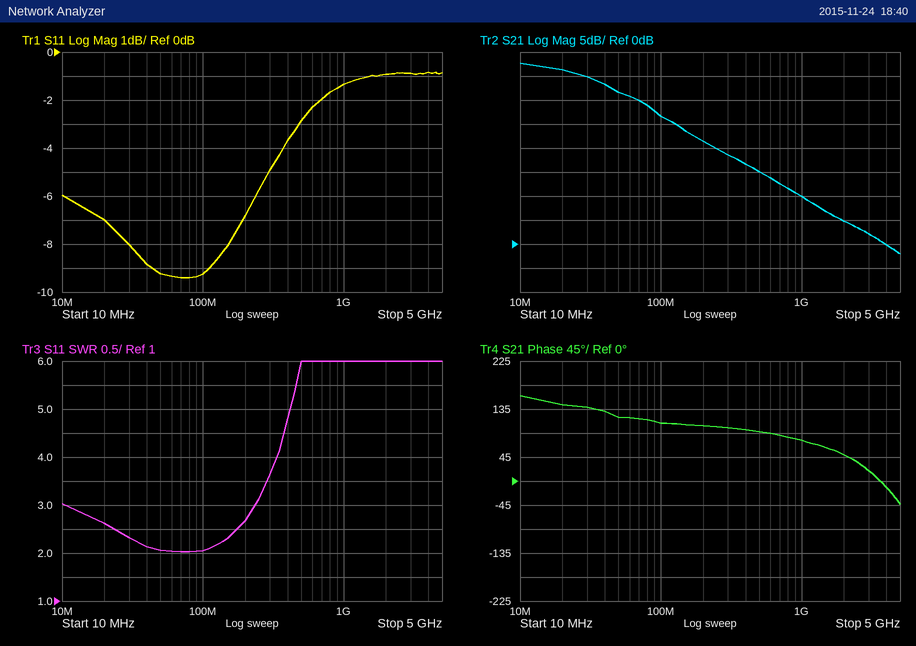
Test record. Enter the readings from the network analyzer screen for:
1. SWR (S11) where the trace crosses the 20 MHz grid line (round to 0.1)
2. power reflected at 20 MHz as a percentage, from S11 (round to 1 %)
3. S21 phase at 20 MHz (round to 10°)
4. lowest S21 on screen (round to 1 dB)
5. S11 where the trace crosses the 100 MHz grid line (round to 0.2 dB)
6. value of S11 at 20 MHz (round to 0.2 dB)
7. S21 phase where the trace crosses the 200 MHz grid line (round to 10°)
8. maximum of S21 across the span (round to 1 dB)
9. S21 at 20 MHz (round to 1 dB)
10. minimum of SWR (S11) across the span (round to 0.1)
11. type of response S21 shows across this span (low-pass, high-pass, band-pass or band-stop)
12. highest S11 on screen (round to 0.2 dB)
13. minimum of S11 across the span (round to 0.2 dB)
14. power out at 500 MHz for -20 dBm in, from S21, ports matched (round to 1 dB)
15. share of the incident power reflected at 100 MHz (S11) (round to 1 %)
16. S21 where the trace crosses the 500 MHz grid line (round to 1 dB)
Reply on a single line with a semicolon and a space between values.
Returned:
2.6; 20 %; 140°; -2 dB; -9.2 dB; -7.0 dB; 100°; 38 dB; 36 dB; 2.0; low-pass; -0.8 dB; -9.4 dB; -5 dBm; 12 %; 15 dB
